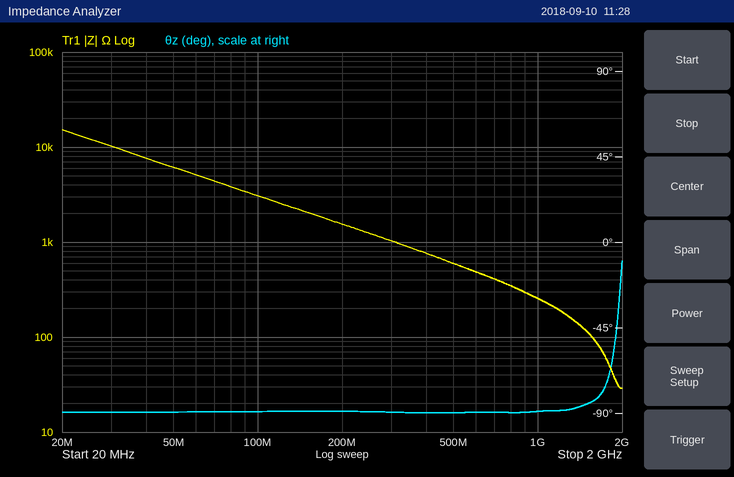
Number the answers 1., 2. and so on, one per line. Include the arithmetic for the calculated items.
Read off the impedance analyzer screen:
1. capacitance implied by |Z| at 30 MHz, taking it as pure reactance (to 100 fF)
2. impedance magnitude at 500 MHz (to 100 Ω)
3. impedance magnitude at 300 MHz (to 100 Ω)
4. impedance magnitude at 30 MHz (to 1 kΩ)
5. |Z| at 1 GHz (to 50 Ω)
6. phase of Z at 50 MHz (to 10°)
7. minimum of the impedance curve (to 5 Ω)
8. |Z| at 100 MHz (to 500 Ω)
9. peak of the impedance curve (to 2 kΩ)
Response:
1. C = 1/(2π × 30 MHz × 10 kΩ) ≈ 531 fF, so 500 fF to the nearest 100 fF
2. 600 Ω
3. 1.0 kΩ
4. 10 kΩ
5. 250 Ω
6. -90°
7. 30 Ω
8. 3.0 kΩ
9. 16 kΩ
